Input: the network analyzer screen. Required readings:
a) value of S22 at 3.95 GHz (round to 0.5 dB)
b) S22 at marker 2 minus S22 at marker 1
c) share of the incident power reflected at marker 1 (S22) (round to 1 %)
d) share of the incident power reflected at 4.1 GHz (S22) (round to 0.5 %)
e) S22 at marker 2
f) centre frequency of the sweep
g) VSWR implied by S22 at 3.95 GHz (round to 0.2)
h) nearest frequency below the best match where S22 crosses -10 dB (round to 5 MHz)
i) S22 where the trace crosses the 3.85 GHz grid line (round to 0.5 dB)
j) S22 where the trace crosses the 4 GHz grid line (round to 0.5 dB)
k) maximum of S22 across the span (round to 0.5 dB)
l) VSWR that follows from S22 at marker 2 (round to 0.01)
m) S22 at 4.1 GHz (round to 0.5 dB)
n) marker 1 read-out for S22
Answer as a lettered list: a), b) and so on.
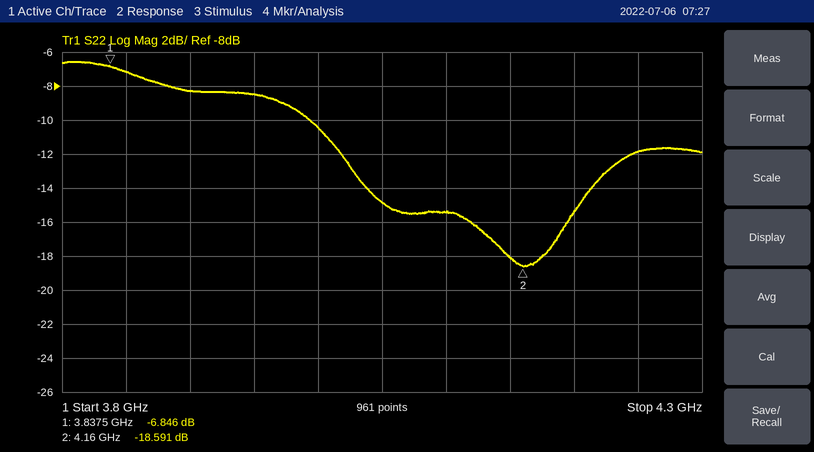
a) -8.5 dB
b) -11.745 dB
c) 21 %
d) 3.0 %
e) -18.591 dB
f) 4.05 GHz
g) 2.2
h) 3.995 GHz
i) -7.0 dB
j) -10.5 dB
k) -6.5 dB
l) 1.27
m) -15.5 dB
n) -6.846 dB
